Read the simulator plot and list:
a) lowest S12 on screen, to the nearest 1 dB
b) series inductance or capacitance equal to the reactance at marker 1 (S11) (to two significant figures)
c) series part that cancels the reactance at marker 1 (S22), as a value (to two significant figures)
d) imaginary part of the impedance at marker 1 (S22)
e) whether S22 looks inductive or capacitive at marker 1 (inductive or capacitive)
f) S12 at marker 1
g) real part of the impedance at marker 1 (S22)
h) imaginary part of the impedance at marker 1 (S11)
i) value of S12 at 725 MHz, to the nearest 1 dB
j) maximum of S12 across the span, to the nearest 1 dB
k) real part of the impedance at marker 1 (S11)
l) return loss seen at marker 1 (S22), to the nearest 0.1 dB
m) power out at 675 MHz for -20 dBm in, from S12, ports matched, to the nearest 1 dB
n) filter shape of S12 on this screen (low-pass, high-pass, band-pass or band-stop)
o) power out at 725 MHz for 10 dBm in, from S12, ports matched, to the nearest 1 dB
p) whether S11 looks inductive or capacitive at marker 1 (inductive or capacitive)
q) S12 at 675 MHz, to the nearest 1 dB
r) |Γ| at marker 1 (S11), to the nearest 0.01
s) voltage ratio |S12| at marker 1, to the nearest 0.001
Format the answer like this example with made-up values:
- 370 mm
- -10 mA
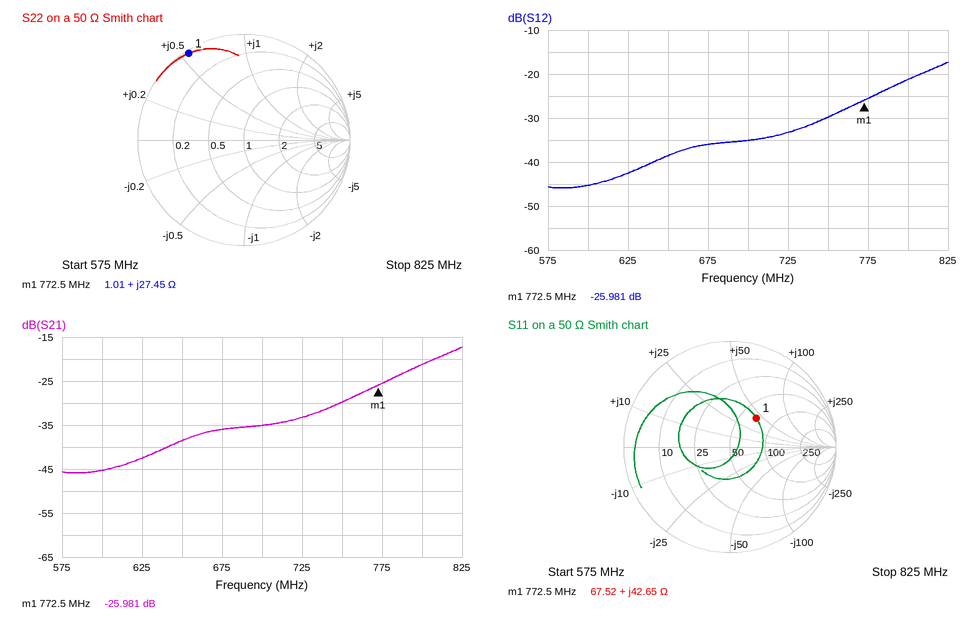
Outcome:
- -46 dB
- 8.8 nH
- 7.5 pF
- +27.45 Ω
- inductive
- -25.981 dB
- 1.01 Ω
- +42.65 Ω
- -33 dB
- -17 dB
- 67.52 Ω
- 0.3 dB
- -56 dBm
- high-pass
- -23 dBm
- inductive
- -36 dB
- 0.37
- 0.050
